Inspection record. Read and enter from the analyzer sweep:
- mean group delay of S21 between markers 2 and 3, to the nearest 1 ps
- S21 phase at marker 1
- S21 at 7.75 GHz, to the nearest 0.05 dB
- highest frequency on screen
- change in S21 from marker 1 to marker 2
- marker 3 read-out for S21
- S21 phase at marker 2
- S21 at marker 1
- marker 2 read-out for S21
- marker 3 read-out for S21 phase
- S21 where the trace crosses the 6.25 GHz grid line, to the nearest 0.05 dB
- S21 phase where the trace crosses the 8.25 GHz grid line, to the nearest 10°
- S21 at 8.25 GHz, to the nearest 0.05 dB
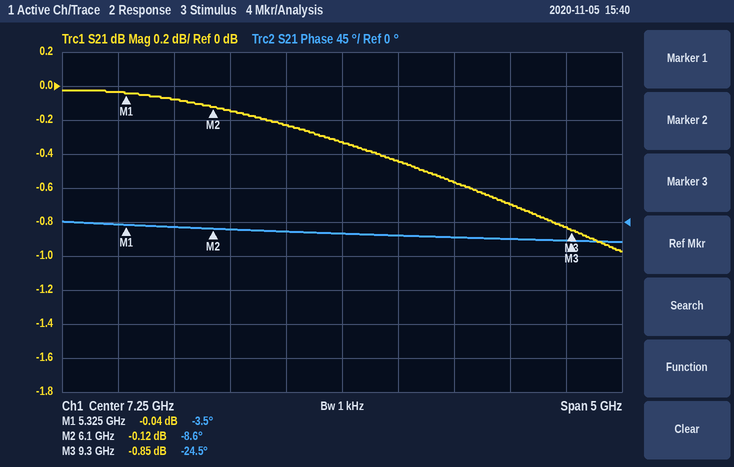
14 ps
-3.5°
-0.45 dB
9.75 GHz
-0.08 dB
-0.85 dB
-8.6°
-0.04 dB
-0.12 dB
-24.5°
-0.15 dB
-20°
-0.55 dB
